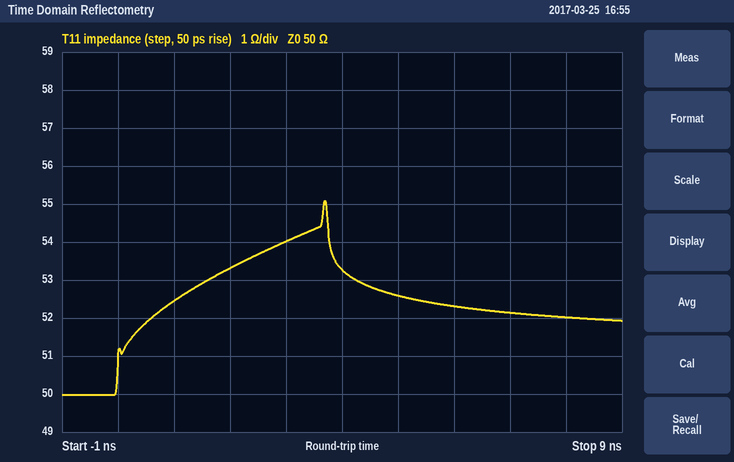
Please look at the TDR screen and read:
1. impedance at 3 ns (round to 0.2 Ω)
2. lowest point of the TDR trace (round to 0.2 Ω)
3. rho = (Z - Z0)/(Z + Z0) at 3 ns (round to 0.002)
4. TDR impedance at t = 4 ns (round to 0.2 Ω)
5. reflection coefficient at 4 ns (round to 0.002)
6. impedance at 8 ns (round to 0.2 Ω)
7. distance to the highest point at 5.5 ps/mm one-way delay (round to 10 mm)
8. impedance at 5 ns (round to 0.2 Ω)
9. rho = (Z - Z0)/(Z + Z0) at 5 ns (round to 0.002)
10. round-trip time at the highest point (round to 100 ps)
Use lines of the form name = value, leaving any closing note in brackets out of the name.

impedance at 3 ns = 54.0 Ω
lowest point of the TDR trace = 50.0 Ω
rho = (Z - Z0)/(Z + Z0) at 3 ns = +0.038
TDR impedance at t = 4 ns = 53.2 Ω
reflection coefficient at 4 ns = +0.032
impedance at 8 ns = 52.0 Ω
distance to the highest point at 5.5 ps/mm one-way delay = 340 mm
impedance at 5 ns = 52.6 Ω
rho = (Z - Z0)/(Z + Z0) at 5 ns = +0.026
round-trip time at the highest point = 3.7 ns
